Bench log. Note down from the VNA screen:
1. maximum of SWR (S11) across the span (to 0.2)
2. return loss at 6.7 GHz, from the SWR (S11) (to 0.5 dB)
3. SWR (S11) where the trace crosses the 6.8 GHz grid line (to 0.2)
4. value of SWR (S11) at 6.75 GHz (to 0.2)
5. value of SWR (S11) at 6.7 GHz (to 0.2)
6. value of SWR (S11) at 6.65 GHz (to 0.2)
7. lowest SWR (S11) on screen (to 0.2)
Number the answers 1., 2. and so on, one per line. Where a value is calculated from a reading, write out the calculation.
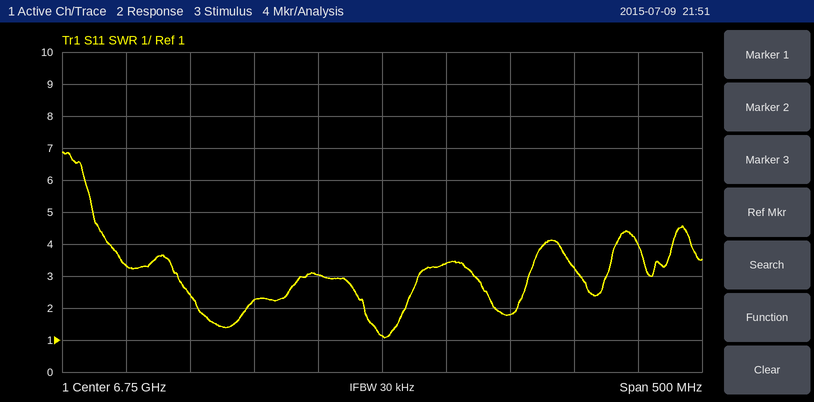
1. 6.8
2. −20 log10((3 − 1)/(3 + 1)) ≈ 6.0 dB
3. 3.4
4. 1.2
5. 3.0
6. 2.2
7. 1.0
